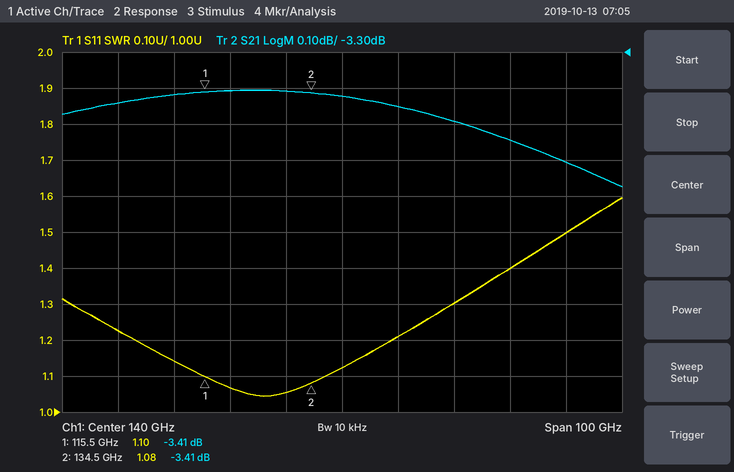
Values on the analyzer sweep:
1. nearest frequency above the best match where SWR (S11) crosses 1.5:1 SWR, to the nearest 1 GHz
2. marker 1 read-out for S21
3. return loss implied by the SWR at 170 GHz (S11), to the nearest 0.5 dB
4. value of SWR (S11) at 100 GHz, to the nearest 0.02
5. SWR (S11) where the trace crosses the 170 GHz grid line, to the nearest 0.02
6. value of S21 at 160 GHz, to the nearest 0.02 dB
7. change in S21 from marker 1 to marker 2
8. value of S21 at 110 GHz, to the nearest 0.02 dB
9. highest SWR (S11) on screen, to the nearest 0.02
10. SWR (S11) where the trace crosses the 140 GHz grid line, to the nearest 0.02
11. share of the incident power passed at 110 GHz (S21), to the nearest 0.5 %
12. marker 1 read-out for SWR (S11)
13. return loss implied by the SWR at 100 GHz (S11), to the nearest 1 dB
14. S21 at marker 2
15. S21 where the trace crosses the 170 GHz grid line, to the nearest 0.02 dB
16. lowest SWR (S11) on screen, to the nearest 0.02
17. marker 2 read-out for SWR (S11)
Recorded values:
180 GHz
-3.41 dB
15.5 dB
1.22
1.40
-3.50 dB
0.00 dB
-3.42 dB
1.60
1.12
45.5 %
1.10
20 dB
-3.41 dB
-3.54 dB
1.04
1.08
